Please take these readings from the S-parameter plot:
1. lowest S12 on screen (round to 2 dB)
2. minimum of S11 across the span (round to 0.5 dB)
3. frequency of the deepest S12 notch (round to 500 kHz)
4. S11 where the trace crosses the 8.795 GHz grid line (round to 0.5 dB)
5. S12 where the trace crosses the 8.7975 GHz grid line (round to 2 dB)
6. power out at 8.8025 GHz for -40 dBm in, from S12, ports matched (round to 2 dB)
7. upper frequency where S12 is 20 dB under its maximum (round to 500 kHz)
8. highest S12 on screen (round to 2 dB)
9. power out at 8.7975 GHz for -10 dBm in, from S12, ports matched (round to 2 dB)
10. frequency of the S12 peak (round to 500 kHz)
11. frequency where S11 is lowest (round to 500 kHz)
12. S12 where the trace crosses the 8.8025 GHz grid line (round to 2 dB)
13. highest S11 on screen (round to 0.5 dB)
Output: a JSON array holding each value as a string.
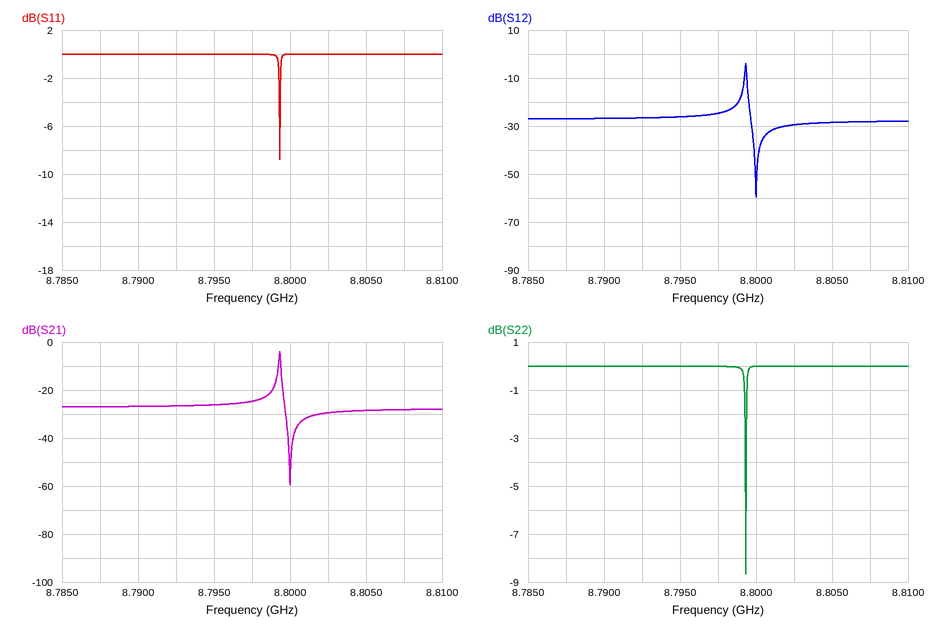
["-60 dB", "-9.0 dB", "8.8000 GHz", "0.0 dB", "-24 dB", "-70 dBm", "8.7995 GHz", "-4 dB", "-34 dBm", "8.7995 GHz", "8.7995 GHz", "-30 dB", "0.0 dB"]
